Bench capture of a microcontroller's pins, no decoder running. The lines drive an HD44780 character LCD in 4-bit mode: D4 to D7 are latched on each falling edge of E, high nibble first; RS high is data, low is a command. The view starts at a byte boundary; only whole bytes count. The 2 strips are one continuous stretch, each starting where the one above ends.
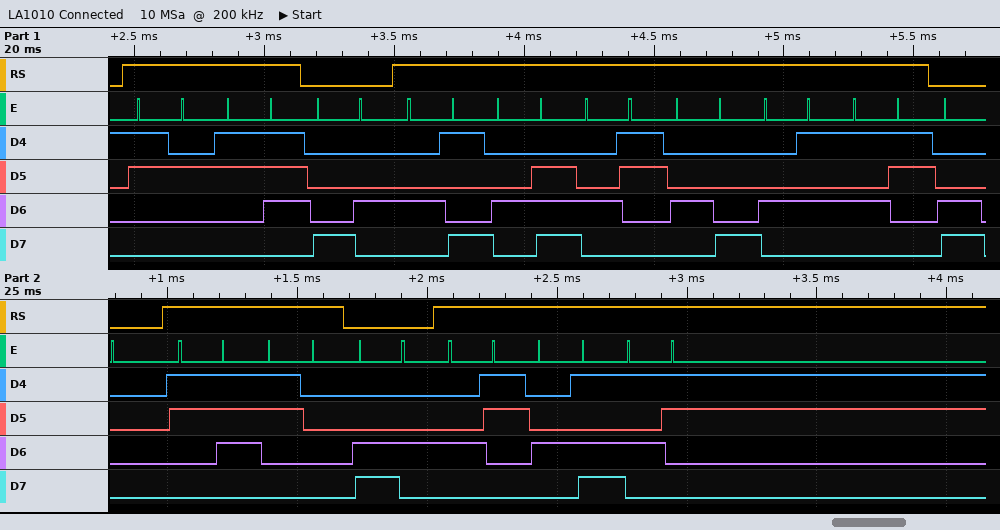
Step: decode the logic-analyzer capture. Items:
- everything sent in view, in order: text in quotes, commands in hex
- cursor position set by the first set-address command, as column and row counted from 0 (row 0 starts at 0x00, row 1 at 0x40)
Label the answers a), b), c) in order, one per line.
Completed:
a) "27" 0x84 "INCHES" 0xC0 "70" 0xC4 "CMS"
b) column 4, row 0
